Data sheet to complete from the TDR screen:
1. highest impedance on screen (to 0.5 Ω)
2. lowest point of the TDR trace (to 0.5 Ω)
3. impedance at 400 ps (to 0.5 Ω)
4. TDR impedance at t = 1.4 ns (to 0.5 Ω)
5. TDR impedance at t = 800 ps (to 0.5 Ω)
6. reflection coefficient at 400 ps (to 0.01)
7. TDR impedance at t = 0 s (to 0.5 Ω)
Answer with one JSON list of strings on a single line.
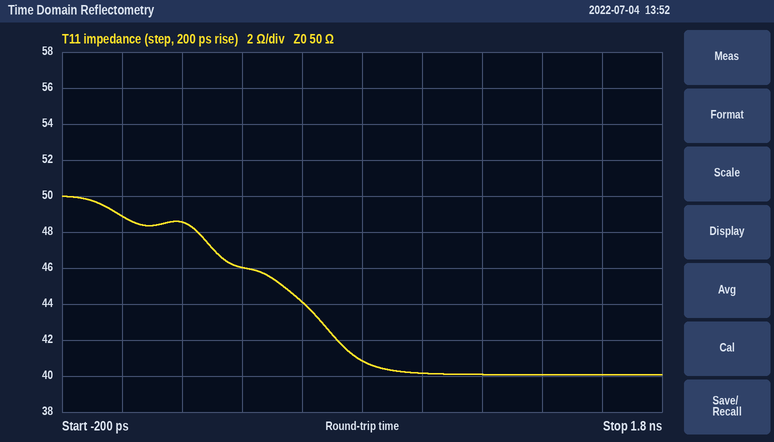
["50.0 Ω", "40.0 Ω", "46.0 Ω", "40.0 Ω", "41.0 Ω", "-0.04", "49.0 Ω"]
